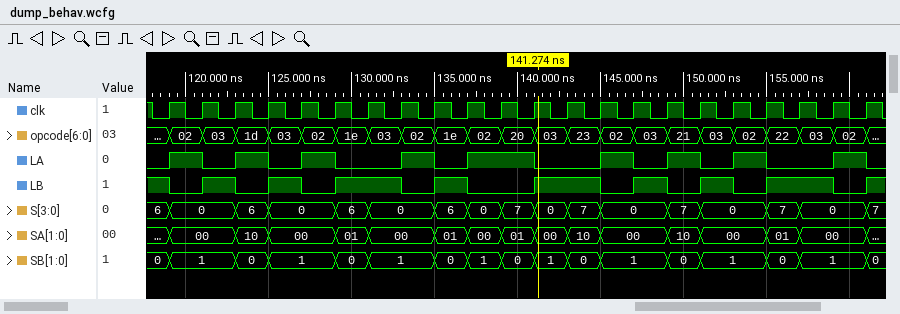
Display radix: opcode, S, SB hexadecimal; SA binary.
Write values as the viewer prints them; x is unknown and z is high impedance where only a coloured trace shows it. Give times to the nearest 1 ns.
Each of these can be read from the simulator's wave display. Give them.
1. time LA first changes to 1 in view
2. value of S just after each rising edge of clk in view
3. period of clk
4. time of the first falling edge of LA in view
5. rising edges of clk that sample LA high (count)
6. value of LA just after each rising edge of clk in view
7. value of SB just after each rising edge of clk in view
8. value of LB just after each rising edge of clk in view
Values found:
119 ns
0, 0, 6, 0, 0, 6, 0, 0, 6, 0, 7, 0, 7, 0, 0, 7, 0, 0, 7, 0, 0, 7
2 ns
121 ns
10
1 0 1 0 1 0 0 1 0 1 1 0 0 1 0 1 0 1 0 0 1 0
1, 1, 0, 1, 1, 0, 1, 1, 0, 1, 0, 1, 0, 1, 1, 0, 1, 1, 0, 1, 1, 0
0 1 0 1 0 1 1 0 1 0 0 1 1 0 1 0 1 0 1 1 0 1
